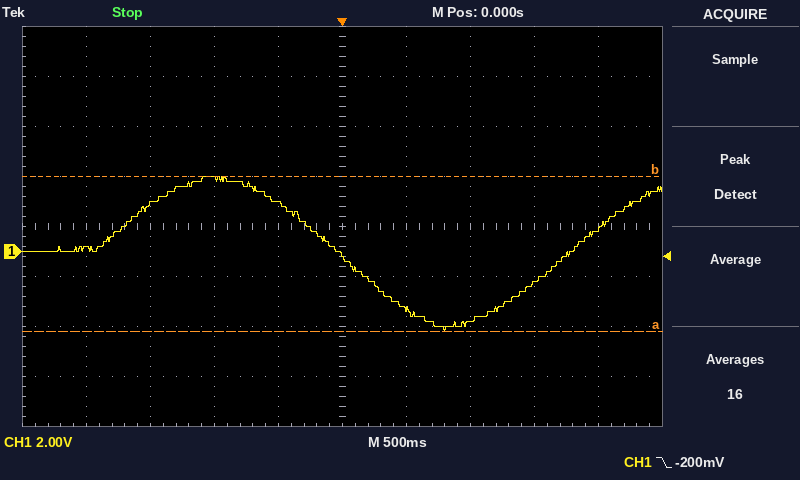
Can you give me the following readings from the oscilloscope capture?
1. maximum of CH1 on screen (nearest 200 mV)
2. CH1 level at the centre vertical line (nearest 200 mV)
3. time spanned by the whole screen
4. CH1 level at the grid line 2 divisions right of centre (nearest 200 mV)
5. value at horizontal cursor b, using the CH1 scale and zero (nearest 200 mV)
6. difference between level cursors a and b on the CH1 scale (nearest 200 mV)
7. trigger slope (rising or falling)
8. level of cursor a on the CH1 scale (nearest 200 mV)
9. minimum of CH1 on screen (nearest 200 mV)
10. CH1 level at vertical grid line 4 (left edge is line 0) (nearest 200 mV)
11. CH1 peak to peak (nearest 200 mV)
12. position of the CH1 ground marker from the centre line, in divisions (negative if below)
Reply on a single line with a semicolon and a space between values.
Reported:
3.0 V; -200 mV; 5 s; -2.8 V; 3.0 V; 6.2 V; falling; -3.2 V; -3.2 V; 2.0 V; 6.2 V; -0.5 div
